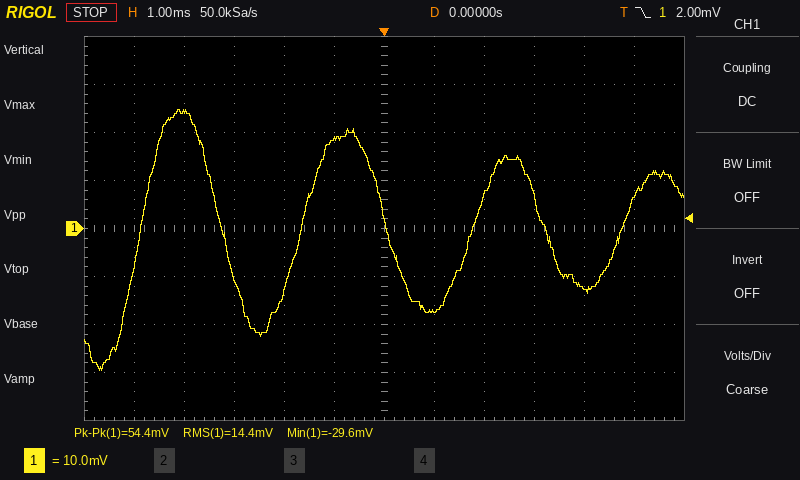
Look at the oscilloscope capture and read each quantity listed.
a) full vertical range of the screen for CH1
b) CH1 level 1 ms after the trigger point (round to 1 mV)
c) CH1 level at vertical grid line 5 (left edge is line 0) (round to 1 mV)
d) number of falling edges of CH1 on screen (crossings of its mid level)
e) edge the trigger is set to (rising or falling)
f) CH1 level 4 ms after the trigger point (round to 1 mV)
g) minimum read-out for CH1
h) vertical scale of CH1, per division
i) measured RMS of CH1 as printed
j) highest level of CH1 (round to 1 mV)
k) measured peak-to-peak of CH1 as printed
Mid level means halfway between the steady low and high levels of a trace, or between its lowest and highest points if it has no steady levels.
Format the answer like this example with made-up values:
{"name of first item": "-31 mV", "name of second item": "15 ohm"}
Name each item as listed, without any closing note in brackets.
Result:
{"full vertical range of the screen for CH1": "80 mV", "CH1 level 1 ms after the trigger point": "-17 mV", "CH1 level at vertical grid line 5 (left edge is line 0)": "19 mV", "number of falling edges of CH1 on screen": "3", "edge the trigger is set to": "falling", "CH1 level 4 ms after the trigger point": "-13 mV", "minimum read-out for CH1": "-29.6 mV", "vertical scale of CH1, per division": "10 mV", "measured RMS of CH1 as printed": "14.4 mV", "highest level of CH1": "25 mV", "measured peak-to-peak of CH1 as printed": "54.4 mV"}
